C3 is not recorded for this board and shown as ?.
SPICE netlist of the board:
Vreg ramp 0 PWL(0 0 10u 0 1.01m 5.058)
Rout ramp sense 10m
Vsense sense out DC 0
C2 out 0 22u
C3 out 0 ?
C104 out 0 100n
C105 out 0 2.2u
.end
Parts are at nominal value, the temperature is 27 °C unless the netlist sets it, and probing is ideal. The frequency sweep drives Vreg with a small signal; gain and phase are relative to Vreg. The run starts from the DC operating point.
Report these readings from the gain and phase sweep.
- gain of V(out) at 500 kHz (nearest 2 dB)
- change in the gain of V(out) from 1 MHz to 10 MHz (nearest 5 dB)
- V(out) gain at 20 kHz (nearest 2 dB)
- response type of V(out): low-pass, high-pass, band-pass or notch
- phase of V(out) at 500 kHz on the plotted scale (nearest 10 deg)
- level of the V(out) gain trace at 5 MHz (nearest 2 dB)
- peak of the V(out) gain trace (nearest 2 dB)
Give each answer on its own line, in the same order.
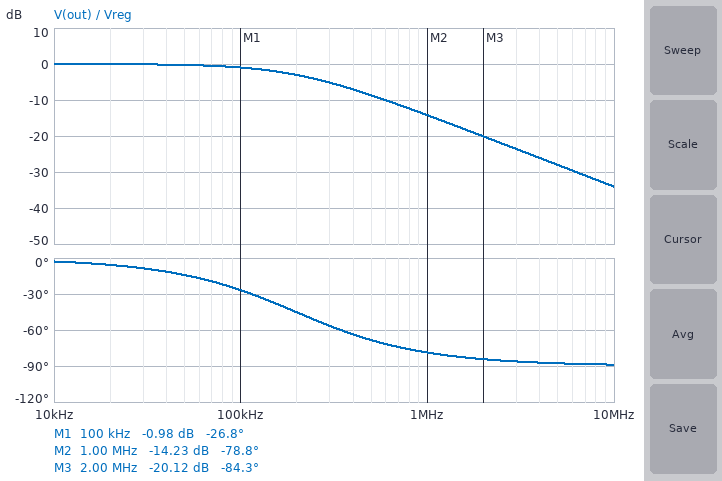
-8 dB
-20 dB
0 dB
low-pass
-70 deg
-28 dB
0 dB
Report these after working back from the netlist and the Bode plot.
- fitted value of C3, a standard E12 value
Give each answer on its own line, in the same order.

56 µF
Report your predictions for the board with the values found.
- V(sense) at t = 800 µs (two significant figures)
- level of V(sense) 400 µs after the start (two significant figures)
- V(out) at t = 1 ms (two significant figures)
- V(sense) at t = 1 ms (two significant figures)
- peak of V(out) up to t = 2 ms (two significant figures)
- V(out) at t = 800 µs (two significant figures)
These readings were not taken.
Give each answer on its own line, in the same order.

4.0 V
2.0 V
5.0 V
5.0 V
5.1 V
4.0 V
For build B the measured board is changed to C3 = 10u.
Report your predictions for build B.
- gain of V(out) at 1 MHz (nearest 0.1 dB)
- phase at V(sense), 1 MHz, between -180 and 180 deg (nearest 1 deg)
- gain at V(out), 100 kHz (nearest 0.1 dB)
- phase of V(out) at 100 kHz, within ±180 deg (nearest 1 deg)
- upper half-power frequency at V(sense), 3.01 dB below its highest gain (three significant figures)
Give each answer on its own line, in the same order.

-7.5 dB
-65 deg
-0.2 dB
-12 deg
464 kHz
